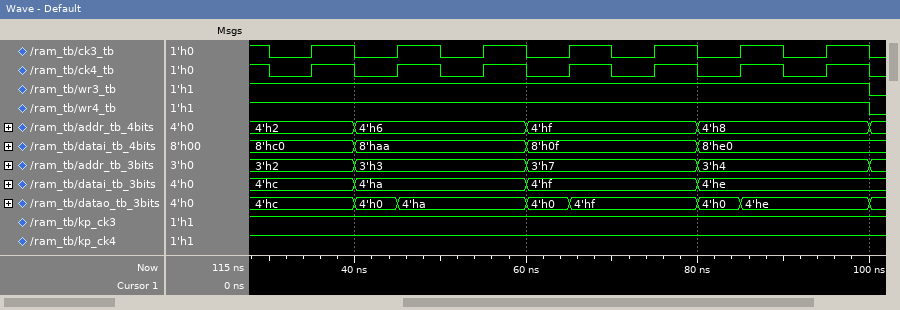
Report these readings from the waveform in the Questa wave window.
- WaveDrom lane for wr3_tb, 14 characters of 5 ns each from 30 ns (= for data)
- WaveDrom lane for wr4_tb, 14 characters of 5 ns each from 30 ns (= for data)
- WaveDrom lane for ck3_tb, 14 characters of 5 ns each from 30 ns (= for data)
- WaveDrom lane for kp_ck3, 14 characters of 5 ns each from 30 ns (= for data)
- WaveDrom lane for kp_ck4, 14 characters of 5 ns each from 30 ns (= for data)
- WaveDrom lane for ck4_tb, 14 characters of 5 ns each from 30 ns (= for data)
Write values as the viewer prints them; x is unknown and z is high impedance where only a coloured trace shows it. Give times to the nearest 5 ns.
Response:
{name: 'wr3_tb', wave: '1.............'}
{name: 'wr4_tb', wave: '1.............'}
{name: 'ck3_tb', wave: '01010101010101'}
{name: 'kp_ck3', wave: '1.............'}
{name: 'kp_ck4', wave: '1.............'}
{name: 'ck4_tb', wave: '01010101010101'}
